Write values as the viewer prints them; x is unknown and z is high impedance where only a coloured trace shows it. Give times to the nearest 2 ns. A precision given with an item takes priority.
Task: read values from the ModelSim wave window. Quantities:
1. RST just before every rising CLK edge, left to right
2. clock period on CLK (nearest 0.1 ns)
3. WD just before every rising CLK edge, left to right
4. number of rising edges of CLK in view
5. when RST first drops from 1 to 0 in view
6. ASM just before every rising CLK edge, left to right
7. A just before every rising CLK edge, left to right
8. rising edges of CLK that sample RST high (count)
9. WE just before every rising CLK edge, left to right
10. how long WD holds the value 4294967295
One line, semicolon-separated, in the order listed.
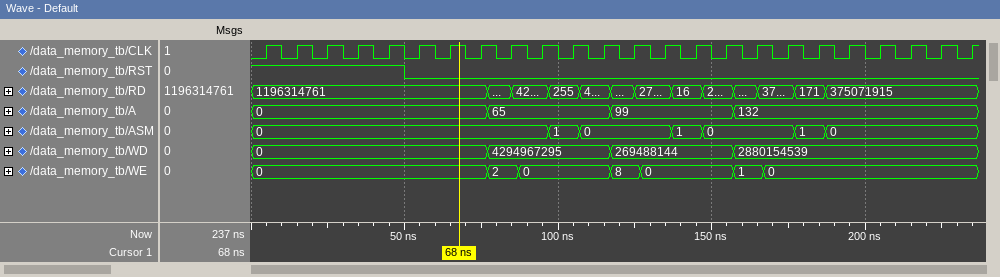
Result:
1 1 1 1 1 0 0 0 0 0 0 0 0 0 0 0 0 0 0 0 0 0 0 0; 10 ns; 0, 0, 0, 0, 0, 0, 0, 0, 4294967295, 4294967295, 4294967295, 4294967295, 269488144, 269488144, 269488144, 269488144, 2880154539, 2880154539, 2880154539, 2880154539, 2880154539, 2880154539, 2880154539, 2880154539; 24; 50 ns; 0, 0, 0, 0, 0, 0, 0, 0, 0, 0, 1, 0, 0, 0, 1, 0, 0, 0, 1, 0, 0, 0, 0, 0; 0, 0, 0, 0, 0, 0, 0, 0, 65, 65, 65, 65, 99, 99, 99, 99, 132, 132, 132, 132, 132, 132, 132, 132; 5; 0, 0, 0, 0, 0, 0, 0, 0, 2, 0, 0, 0, 8, 0, 0, 0, 1, 0, 0, 0, 0, 0, 0, 0; 40 ns
